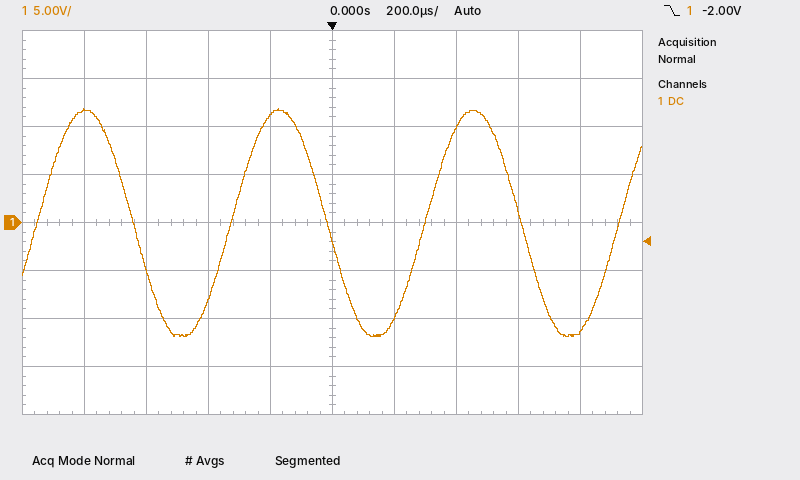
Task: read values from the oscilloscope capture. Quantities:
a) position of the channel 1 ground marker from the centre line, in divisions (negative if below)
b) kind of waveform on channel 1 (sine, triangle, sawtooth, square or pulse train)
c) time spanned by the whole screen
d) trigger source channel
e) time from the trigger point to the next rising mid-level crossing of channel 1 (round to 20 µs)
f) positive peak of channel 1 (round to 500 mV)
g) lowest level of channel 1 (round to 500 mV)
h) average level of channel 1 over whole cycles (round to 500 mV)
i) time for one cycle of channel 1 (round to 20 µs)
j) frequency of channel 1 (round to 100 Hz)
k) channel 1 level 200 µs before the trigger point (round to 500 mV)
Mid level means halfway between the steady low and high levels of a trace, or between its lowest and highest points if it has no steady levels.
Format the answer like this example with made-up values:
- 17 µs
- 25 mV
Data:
- 0.0 div
- sine
- 2 ms
- channel 1
- 300 µs
- 12.0 V
- -12.0 V
- 0.0 V
- 620 µs
- 1.6 kHz
- 11.0 V
